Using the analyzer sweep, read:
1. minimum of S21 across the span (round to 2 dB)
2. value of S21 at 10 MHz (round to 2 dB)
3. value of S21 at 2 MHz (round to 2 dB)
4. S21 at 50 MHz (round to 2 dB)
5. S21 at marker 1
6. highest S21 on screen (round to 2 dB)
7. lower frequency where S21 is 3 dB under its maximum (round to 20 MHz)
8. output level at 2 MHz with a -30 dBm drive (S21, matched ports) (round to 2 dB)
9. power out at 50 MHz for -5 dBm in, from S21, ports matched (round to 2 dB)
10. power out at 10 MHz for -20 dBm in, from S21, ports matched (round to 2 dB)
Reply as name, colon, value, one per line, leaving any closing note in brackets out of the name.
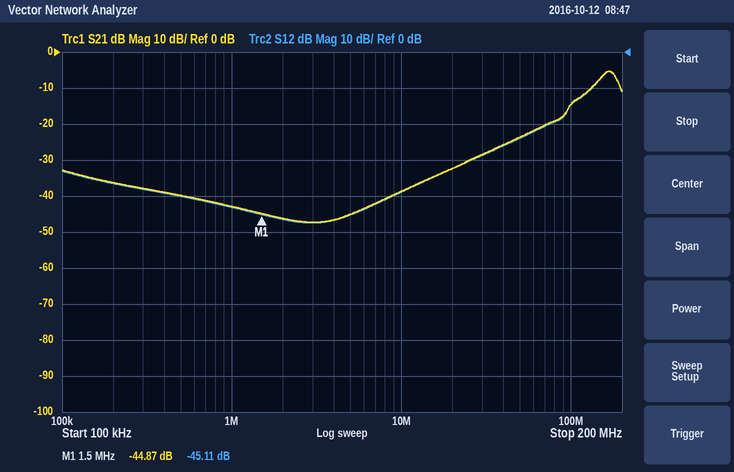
minimum of S21 across the span: -48 dB
value of S21 at 10 MHz: -38 dB
value of S21 at 2 MHz: -46 dB
S21 at 50 MHz: -24 dB
S21 at marker 1: -44.87 dB
highest S21 on screen: -6 dB
lower frequency where S21 is 3 dB under its maximum: 140 MHz
output level at 2 MHz with a -30 dBm drive (S21, matched ports): -76 dBm
power out at 50 MHz for -5 dBm in, from S21, ports matched: -28 dBm
power out at 10 MHz for -20 dBm in, from S21, ports matched: -58 dBm
